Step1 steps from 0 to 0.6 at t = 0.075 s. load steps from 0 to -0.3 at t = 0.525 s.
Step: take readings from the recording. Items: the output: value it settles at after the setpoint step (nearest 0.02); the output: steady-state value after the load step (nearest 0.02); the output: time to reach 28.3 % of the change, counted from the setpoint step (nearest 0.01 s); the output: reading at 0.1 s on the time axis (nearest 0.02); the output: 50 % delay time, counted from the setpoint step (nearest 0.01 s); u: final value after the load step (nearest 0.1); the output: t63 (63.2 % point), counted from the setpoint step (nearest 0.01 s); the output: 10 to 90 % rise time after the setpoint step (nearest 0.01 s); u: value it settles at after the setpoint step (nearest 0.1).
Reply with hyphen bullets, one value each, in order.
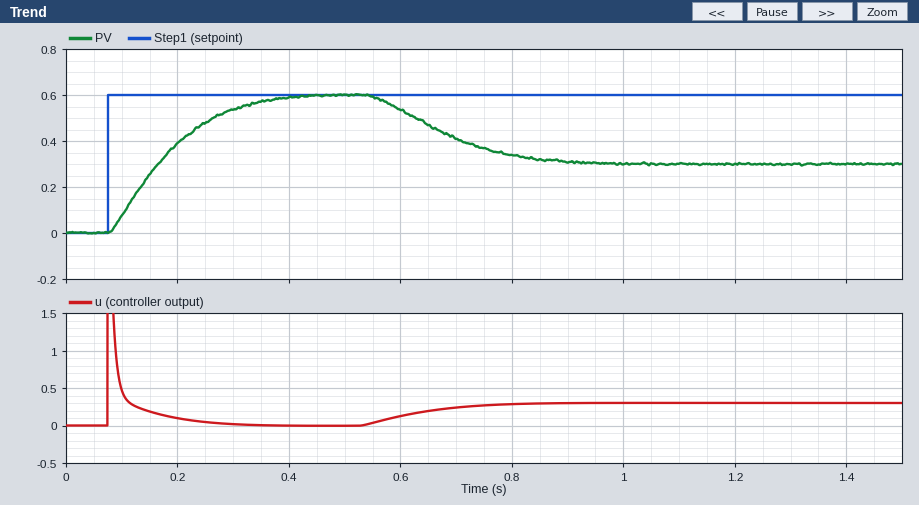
- 0.60
- 0.30
- 0.05 s
- 0.08
- 0.09 s
- 0.3
- 0.12 s
- 0.21 s
- 0.0
